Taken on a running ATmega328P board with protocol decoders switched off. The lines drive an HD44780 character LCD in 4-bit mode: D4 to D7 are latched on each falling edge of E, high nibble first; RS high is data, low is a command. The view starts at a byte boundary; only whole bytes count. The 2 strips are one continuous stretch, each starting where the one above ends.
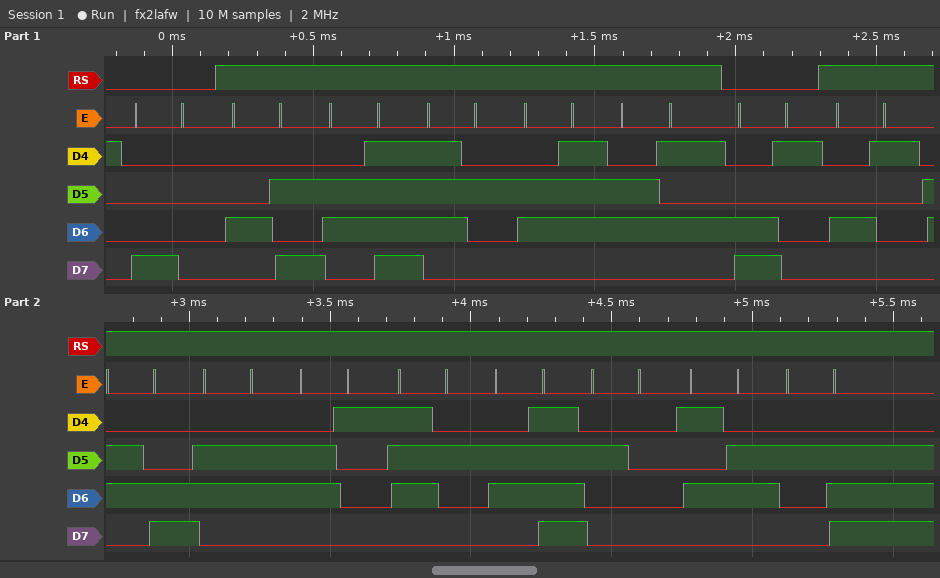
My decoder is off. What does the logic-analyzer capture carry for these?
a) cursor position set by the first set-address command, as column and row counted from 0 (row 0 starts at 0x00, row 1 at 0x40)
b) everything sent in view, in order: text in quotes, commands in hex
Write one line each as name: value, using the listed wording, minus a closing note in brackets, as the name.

cursor position set by the first set-address command, as column and row counted from 0: column 0, row 0
everything sent in view, in order: text in quotes, commands in hex: 0x80 "Jorge" 0xC1 "Alfaro V."
